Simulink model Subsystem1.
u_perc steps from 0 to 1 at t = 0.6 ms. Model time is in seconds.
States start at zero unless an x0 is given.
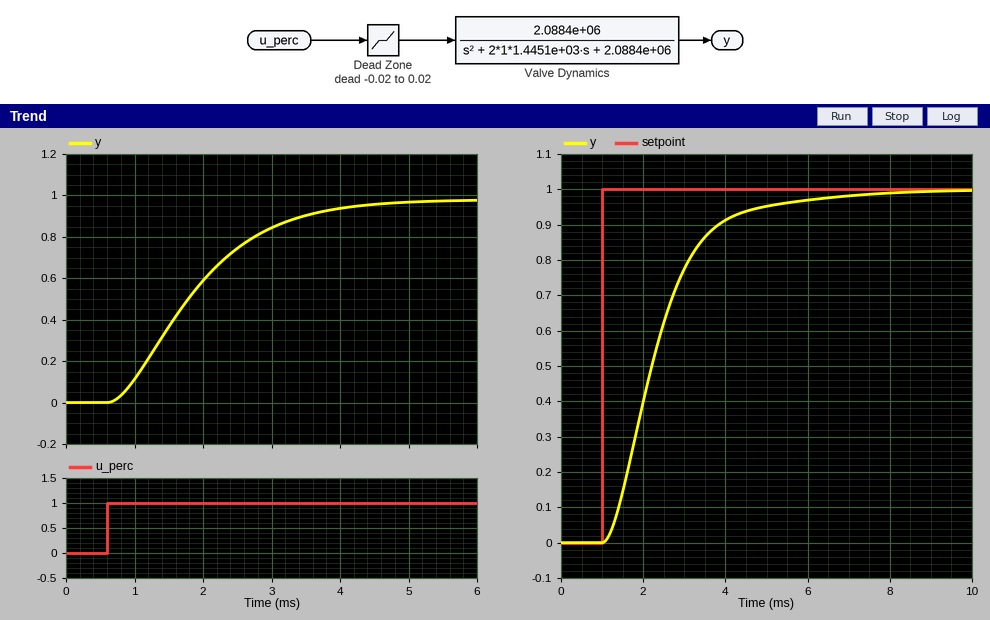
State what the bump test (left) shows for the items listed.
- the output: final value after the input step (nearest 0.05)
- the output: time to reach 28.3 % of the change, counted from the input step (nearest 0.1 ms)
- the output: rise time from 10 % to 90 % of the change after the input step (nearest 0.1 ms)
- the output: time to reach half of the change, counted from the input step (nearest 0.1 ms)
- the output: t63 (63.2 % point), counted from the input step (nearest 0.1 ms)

1.00
0.7 ms
2.3 ms
1.2 ms
1.5 ms
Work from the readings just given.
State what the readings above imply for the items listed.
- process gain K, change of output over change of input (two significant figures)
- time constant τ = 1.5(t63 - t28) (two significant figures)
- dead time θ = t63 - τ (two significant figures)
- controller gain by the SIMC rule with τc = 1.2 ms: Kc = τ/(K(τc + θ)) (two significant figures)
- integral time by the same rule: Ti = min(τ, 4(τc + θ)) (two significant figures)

1.0
1.2 ms
0.30 ms
0.80
1.2 ms
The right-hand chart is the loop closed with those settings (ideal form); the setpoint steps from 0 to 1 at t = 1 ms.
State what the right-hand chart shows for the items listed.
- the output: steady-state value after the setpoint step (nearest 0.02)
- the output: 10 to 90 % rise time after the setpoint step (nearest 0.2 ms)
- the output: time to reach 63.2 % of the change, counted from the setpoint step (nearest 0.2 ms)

1.00
2.4 ms
1.6 ms
